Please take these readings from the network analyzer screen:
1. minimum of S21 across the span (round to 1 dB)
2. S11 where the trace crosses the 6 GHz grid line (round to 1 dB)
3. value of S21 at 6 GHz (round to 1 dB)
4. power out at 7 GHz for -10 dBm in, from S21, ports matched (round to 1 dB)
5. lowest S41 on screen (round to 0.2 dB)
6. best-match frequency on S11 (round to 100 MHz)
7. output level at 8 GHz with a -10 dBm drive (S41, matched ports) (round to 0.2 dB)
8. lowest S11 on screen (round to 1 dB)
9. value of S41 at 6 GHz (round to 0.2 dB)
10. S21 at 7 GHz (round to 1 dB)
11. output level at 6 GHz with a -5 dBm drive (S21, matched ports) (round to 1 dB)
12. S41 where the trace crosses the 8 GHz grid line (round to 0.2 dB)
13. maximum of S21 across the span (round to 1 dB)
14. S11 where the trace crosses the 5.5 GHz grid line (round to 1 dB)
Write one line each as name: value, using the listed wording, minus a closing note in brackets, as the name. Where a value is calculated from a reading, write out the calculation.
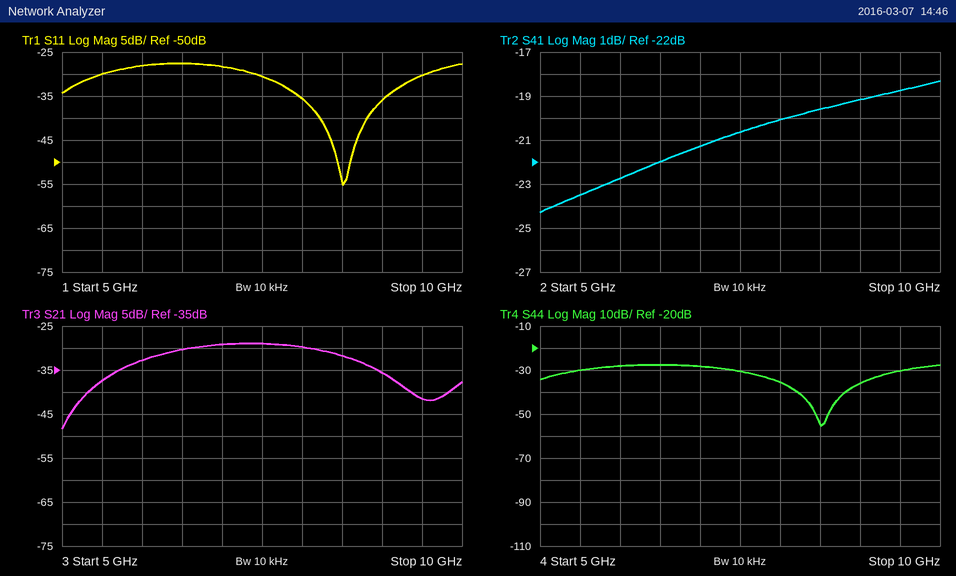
minimum of S21 across the span: -48 dB
S11 where the trace crosses the 6 GHz grid line: -28 dB
value of S21 at 6 GHz: -33 dB
power out at 7 GHz for -10 dBm in, from S21, ports matched: -10 dBm + (-29 dB) = -39 dBm
lowest S41 on screen: -24.2 dB
best-match frequency on S11: 8.5 GHz
output level at 8 GHz with a -10 dBm drive (S41, matched ports): -10 dBm + (-20.0 dB) = -30.0 dBm
lowest S11 on screen: -55 dB
value of S41 at 6 GHz: -22.8 dB
S21 at 7 GHz: -29 dB
output level at 6 GHz with a -5 dBm drive (S21, matched ports): -5 dBm + (-33 dB) = -38 dBm
S41 where the trace crosses the 8 GHz grid line: -20.0 dB
maximum of S21 across the span: -29 dB
S11 where the trace crosses the 5.5 GHz grid line: -30 dB
